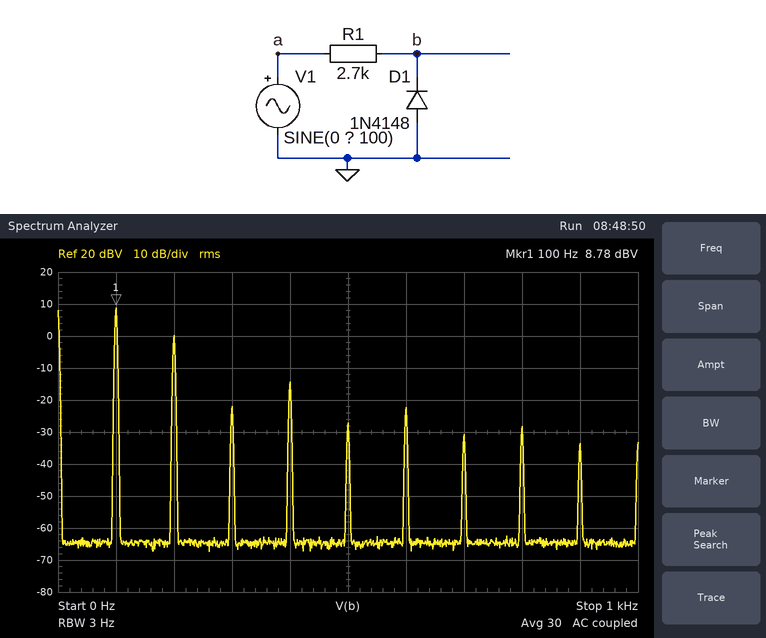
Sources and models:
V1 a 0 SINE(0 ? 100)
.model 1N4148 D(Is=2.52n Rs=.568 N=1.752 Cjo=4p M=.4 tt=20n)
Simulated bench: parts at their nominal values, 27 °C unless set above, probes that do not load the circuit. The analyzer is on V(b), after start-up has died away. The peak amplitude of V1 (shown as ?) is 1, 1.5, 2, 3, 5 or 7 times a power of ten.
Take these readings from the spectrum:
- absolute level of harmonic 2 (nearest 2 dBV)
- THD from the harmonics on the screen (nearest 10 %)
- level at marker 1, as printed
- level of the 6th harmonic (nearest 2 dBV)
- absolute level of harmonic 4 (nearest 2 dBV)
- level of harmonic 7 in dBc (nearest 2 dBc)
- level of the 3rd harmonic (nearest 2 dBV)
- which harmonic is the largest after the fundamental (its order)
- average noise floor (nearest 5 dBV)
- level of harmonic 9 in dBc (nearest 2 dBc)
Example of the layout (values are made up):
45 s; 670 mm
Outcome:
0 dBV; 40 %; 8.78 dBV; -22 dBV; -14 dBV; -40 dBc; -22 dBV; 2; -65 dBV; -42 dBc
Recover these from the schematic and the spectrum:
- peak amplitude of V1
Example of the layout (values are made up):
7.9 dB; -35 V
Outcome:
7 V
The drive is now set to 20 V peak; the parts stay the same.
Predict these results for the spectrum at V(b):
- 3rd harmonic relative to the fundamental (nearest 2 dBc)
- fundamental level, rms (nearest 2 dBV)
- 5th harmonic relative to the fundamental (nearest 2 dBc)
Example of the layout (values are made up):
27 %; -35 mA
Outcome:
-38 dBc; 18 dBV; -44 dBc
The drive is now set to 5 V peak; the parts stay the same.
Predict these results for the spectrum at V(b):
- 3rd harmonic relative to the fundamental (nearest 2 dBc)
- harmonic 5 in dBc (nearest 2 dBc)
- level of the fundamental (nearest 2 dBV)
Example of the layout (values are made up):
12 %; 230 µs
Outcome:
-28 dBc; -34 dBc; 6 dBV
